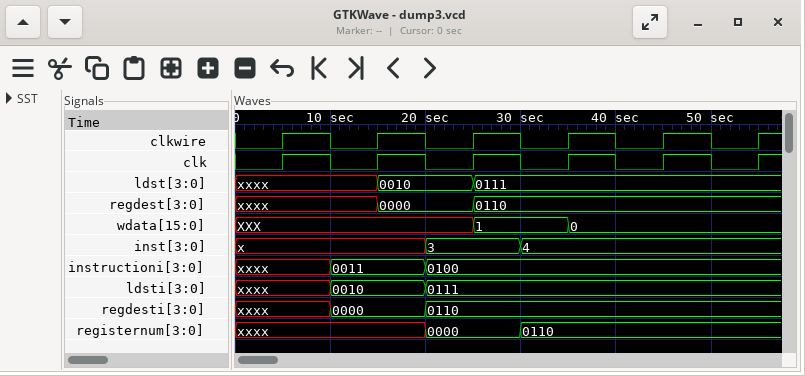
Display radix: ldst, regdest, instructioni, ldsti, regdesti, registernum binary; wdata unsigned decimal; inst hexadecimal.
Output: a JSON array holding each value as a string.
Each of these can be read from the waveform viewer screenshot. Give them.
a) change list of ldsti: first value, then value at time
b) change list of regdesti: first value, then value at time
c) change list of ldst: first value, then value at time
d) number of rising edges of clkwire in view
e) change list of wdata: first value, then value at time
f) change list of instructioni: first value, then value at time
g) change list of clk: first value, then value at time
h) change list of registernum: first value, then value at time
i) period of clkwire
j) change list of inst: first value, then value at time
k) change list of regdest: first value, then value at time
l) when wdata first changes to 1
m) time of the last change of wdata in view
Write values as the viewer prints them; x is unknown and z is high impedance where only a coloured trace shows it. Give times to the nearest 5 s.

["xxxx, 0010 at 10 s, 0111 at 20 s", "xxxx, 0000 at 10 s, 0110 at 20 s", "xxxx, 0010 at 15 s, 0111 at 25 s", "6", "XXX, 1 at 25 s, 0 at 35 s", "xxxx, 0011 at 10 s, 0100 at 20 s", "0, 1 at 5 s, 0 at 10 s, 1 at 15 s, 0 at 20 s, 1 at 25 s, 0 at 30 s, 1 at 35 s, 0 at 40 s, 1 at 45 s, 0 at 50 s, 1 at 55 s", "xxxx, 0000 at 20 s, 0110 at 30 s", "10 s", "x, 3 at 20 s, 4 at 30 s", "xxxx, 0000 at 15 s, 0110 at 25 s", "25 s", "35 s"]
